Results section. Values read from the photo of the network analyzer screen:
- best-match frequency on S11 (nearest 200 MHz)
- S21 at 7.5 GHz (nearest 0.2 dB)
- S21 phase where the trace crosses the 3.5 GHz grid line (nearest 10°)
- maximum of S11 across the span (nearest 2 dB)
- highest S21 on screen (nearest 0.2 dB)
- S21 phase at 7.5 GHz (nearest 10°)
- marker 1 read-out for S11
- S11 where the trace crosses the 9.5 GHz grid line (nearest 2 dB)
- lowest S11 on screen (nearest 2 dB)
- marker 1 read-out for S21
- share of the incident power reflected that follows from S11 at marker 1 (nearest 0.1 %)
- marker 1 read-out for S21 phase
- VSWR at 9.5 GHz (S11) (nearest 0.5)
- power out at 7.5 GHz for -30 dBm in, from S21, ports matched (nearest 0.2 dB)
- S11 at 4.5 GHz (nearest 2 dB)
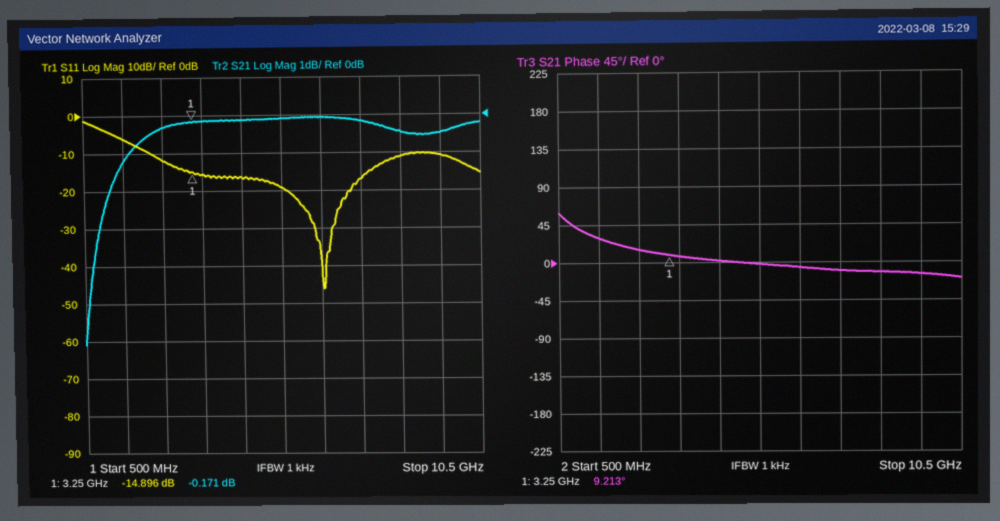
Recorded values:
6.6 GHz
-0.2 dB
10°
-2 dB
0.0 dB
-10°
-14.896 dB
-10 dB
-46 dB
-0.171 dB
3.2 %
9.213°
2.0
-30.2 dBm
-16 dB
